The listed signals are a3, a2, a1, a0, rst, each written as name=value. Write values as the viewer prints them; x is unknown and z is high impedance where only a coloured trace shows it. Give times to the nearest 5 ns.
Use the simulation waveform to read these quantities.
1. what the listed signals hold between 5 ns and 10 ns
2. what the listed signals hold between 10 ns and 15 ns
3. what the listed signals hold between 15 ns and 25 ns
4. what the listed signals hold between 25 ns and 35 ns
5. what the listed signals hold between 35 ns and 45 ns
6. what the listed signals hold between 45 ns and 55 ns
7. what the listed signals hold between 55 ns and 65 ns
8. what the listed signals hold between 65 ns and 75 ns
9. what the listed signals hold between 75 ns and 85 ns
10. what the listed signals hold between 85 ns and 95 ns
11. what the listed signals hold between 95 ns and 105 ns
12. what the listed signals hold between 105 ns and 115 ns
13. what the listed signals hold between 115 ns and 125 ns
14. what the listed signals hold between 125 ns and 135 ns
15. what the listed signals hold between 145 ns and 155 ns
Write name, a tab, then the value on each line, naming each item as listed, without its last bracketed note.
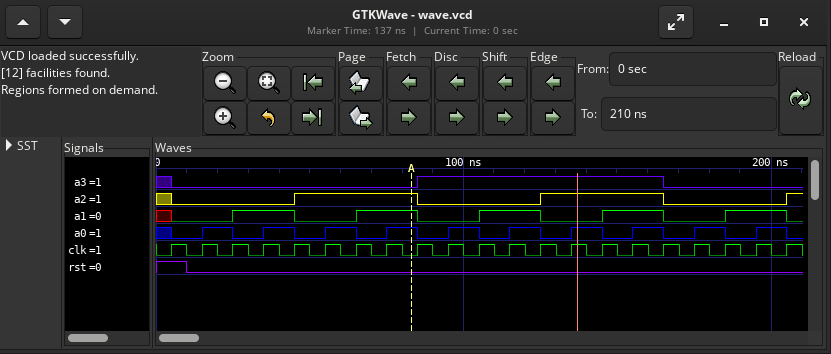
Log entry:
what the listed signals hold between 5 ns and 10 ns	a3=0, a2=0, a1=0, a0=0, rst=1
what the listed signals hold between 10 ns and 15 ns	a3=0, a2=0, a1=0, a0=0, rst=0
what the listed signals hold between 15 ns and 25 ns	a3=0, a2=0, a1=0, a0=1, rst=0
what the listed signals hold between 25 ns and 35 ns	a3=0, a2=0, a1=1, a0=0, rst=0
what the listed signals hold between 35 ns and 45 ns	a3=0, a2=0, a1=1, a0=1, rst=0
what the listed signals hold between 45 ns and 55 ns	a3=0, a2=1, a1=0, a0=0, rst=0
what the listed signals hold between 55 ns and 65 ns	a3=0, a2=1, a1=0, a0=1, rst=0
what the listed signals hold between 65 ns and 75 ns	a3=0, a2=1, a1=1, a0=0, rst=0
what the listed signals hold between 75 ns and 85 ns	a3=0, a2=1, a1=1, a0=1, rst=0
what the listed signals hold between 85 ns and 95 ns	a3=1, a2=0, a1=0, a0=0, rst=0
what the listed signals hold between 95 ns and 105 ns	a3=1, a2=0, a1=0, a0=1, rst=0
what the listed signals hold between 105 ns and 115 ns	a3=1, a2=0, a1=1, a0=0, rst=0
what the listed signals hold between 115 ns and 125 ns	a3=1, a2=0, a1=1, a0=1, rst=0
what the listed signals hold between 125 ns and 135 ns	a3=1, a2=1, a1=0, a0=0, rst=0
what the listed signals hold between 145 ns and 155 ns	a3=1, a2=1, a1=1, a0=0, rst=0
